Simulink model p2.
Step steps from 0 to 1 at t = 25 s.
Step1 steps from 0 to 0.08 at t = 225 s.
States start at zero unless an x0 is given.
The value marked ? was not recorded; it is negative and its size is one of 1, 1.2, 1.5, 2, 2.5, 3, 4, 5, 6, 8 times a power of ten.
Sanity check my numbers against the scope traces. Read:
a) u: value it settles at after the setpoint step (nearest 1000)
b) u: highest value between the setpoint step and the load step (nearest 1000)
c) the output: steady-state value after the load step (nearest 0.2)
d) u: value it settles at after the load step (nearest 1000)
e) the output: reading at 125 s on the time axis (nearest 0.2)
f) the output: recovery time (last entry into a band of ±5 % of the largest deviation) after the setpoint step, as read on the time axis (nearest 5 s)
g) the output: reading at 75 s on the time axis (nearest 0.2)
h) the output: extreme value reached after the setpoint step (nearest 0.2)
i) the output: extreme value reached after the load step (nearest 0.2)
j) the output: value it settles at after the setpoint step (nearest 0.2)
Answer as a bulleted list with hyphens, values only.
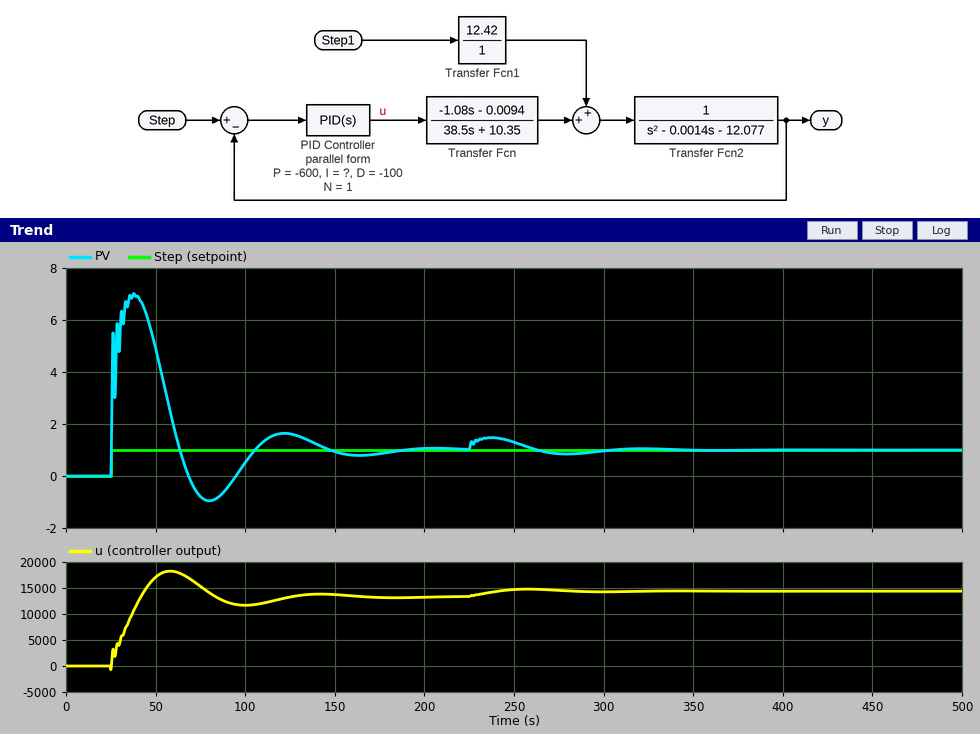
- 13000
- 18000
- 1.0
- 14000
- 1.6
- 135 s
- -0.8
- 7.0
- 1.4
- 1.0
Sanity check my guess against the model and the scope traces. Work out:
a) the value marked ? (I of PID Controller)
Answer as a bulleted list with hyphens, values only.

- -120
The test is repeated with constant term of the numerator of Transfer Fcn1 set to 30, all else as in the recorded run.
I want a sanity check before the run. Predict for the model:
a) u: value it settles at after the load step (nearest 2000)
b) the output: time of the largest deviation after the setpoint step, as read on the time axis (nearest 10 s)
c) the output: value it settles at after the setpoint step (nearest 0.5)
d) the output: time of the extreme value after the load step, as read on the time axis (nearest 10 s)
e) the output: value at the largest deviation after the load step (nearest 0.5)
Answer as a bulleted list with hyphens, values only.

- 16000
- 40 s
- 1.0
- 240 s
- 2.0
